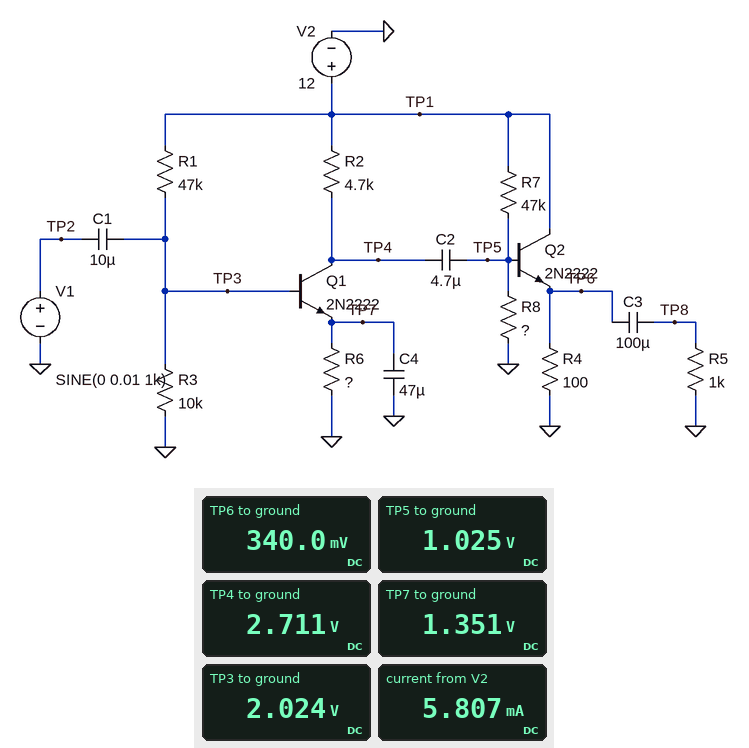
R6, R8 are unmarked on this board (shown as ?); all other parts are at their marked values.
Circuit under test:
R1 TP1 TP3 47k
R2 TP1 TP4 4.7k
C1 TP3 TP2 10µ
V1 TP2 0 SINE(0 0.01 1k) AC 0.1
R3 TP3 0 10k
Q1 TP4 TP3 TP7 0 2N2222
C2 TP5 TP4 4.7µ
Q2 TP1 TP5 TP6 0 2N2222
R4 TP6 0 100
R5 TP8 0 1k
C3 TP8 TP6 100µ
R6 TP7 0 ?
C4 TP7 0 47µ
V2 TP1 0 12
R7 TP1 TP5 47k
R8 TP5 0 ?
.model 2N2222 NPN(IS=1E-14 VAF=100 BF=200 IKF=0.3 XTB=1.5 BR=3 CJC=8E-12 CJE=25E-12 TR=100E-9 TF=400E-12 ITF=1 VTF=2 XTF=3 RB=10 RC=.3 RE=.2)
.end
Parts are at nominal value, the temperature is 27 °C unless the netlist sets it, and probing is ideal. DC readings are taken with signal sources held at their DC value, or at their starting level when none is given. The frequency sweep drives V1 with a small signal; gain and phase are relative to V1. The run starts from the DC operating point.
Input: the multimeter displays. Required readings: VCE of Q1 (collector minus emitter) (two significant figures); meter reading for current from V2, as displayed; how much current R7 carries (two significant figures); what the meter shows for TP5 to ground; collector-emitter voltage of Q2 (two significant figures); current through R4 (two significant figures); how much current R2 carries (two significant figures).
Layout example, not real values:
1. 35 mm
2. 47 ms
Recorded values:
1. 1.4 V
2. 5.807 mA
3. 230 µA
4. 1.025 V
5. 12 V
6. 3.4 mA
7. 2.0 mA
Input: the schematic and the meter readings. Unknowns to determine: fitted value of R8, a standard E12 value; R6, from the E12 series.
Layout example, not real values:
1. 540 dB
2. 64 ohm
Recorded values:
1. 4.7 kΩ
2. 680 Ω
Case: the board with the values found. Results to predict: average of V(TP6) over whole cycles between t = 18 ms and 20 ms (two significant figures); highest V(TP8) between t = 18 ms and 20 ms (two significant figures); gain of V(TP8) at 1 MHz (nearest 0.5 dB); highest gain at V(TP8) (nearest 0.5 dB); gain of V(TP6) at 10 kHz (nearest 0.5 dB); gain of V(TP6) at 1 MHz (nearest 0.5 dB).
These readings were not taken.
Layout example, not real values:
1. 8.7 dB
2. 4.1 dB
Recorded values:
1. 620 mV
2. 1.2 V
3. 42.0 dB
4. 42.5 dB
5. 42.5 dB
6. 42.0 dB
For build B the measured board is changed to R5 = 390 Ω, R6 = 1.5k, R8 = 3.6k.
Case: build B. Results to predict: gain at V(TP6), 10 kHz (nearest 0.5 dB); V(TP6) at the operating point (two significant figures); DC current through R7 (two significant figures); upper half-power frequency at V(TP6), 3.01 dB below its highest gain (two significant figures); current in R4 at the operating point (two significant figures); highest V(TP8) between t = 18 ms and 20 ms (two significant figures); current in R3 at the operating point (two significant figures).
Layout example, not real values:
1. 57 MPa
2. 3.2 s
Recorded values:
1. 34.5 dB
2. 160 mV
3. 240 µA
4. 4.6 MHz
5. 1.6 mA
6. 470 mV
7. 210 µA
